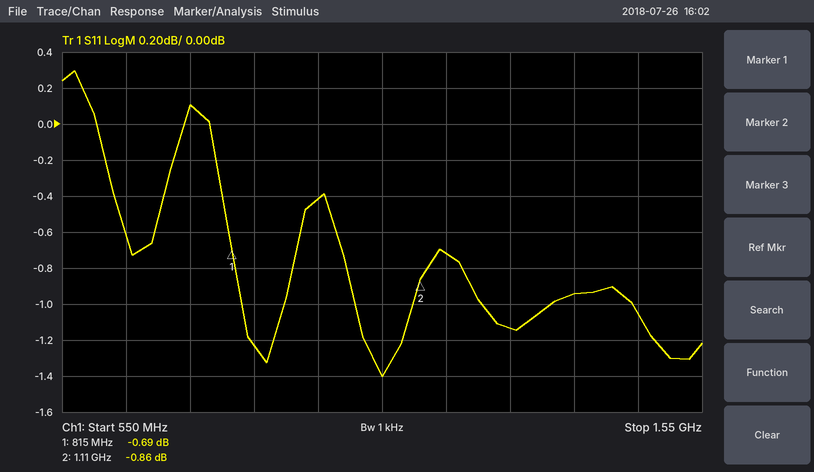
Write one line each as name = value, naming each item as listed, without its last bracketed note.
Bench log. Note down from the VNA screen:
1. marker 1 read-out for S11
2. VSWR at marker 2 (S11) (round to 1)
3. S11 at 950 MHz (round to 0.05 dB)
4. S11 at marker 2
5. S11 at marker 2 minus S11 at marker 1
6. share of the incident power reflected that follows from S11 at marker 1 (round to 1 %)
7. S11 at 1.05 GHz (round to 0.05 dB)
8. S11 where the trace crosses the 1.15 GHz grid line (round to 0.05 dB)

marker 1 read-out for S11 = -0.69 dB
VSWR at marker 2 (S11) = 20
S11 at 950 MHz = -0.40 dB
S11 at marker 2 = -0.86 dB
S11 at marker 2 minus S11 at marker 1 = -0.17 dB
share of the incident power reflected that follows from S11 at marker 1 = 85 %
S11 at 1.05 GHz = -1.40 dB
S11 where the trace crosses the 1.15 GHz grid line = -0.70 dB
